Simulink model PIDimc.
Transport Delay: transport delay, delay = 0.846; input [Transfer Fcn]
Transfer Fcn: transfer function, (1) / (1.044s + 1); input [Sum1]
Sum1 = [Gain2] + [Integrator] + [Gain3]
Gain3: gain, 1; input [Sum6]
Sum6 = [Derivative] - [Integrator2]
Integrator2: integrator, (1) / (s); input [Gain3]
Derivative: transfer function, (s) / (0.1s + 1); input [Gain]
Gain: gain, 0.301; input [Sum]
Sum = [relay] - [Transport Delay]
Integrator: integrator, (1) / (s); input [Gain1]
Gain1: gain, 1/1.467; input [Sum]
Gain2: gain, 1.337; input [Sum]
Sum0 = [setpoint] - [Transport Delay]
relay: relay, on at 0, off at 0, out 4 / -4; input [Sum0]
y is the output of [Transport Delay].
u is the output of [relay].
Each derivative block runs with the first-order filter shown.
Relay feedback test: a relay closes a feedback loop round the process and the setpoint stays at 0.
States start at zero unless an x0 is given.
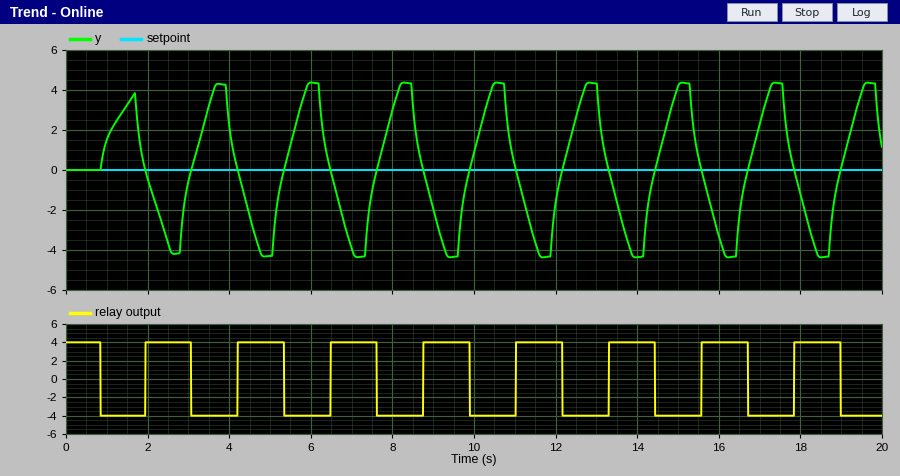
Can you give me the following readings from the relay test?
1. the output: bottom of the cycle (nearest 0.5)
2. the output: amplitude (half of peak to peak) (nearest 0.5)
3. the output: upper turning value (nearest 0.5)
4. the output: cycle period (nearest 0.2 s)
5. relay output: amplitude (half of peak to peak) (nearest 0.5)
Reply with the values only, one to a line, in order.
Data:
-4.5
4.5
4.5
2.2 s
4.0
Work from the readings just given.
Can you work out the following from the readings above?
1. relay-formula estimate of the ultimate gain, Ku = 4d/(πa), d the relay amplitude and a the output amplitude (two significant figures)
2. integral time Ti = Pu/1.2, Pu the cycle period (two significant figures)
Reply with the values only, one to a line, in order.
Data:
1.1
1.8 s
